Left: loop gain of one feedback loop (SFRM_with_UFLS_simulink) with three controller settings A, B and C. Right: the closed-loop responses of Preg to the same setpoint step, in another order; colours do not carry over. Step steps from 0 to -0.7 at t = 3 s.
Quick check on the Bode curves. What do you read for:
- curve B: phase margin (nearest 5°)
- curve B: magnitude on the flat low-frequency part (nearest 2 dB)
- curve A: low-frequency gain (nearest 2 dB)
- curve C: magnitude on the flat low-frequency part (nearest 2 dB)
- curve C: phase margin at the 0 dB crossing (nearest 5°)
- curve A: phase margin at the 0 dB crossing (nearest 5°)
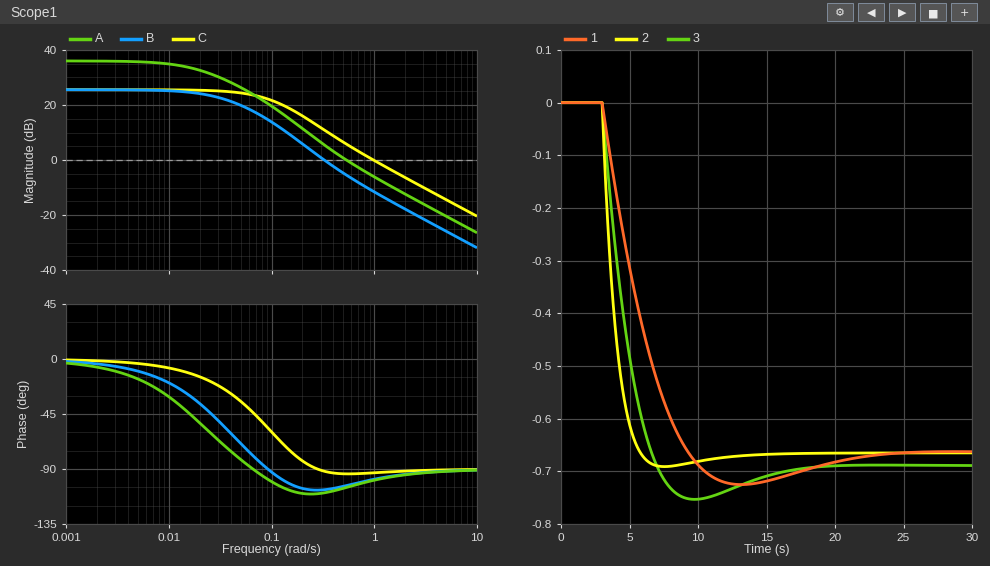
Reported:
75°
26 dB
36 dB
26 dB
85°
75°
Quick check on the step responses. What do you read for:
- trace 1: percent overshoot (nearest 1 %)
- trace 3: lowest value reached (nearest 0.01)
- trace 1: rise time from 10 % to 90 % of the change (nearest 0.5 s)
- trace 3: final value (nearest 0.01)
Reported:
9 %
-0.75
4.5 s
-0.69
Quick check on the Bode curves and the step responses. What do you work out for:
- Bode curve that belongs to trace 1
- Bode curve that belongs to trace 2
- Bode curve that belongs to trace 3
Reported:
B
C
A
